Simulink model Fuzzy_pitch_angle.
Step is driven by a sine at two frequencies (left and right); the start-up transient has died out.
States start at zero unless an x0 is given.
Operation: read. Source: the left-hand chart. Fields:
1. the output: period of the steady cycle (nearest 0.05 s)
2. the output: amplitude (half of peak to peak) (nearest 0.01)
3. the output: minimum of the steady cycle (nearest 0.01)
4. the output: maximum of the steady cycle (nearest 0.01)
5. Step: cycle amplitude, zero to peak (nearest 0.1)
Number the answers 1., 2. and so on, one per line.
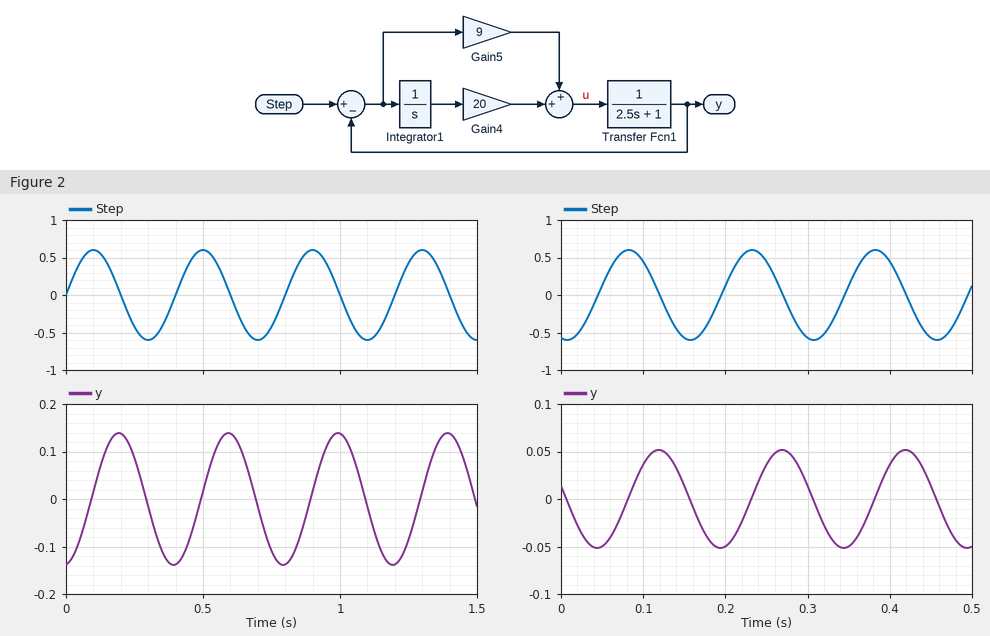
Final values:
1. 0.40 s
2. 0.14
3. -0.14
4. 0.14
5. 0.6
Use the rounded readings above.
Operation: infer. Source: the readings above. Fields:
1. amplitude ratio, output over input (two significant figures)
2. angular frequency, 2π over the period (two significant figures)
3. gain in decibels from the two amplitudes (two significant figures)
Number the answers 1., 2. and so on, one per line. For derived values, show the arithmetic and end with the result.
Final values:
1. 0.14 / 0.6 = 0.23
2. 2π / 0.4 = 16 rad/s
3. 20 log10(0.14 / 0.6) = -13 dB
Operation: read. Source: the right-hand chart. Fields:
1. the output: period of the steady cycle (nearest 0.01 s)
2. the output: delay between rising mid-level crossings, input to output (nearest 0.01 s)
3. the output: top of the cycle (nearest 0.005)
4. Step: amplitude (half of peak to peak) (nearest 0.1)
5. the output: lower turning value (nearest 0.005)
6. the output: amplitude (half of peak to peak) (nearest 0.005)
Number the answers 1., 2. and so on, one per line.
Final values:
1. 0.15 s
2. 0.04 s
3. 0.050
4. 0.6
5. -0.050
6. 0.050
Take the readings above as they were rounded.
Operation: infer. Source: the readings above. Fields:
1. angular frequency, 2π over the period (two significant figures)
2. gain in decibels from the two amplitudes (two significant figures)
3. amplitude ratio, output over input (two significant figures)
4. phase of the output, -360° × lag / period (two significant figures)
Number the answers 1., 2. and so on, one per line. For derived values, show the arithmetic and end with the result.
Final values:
1. 2π / 0.15 = 42 rad/s
2. 20 log10(0.05 / 0.6) = -22 dB
3. 0.05 / 0.6 = 0.083
4. -360 × 0.04 / 0.15 = -96°
